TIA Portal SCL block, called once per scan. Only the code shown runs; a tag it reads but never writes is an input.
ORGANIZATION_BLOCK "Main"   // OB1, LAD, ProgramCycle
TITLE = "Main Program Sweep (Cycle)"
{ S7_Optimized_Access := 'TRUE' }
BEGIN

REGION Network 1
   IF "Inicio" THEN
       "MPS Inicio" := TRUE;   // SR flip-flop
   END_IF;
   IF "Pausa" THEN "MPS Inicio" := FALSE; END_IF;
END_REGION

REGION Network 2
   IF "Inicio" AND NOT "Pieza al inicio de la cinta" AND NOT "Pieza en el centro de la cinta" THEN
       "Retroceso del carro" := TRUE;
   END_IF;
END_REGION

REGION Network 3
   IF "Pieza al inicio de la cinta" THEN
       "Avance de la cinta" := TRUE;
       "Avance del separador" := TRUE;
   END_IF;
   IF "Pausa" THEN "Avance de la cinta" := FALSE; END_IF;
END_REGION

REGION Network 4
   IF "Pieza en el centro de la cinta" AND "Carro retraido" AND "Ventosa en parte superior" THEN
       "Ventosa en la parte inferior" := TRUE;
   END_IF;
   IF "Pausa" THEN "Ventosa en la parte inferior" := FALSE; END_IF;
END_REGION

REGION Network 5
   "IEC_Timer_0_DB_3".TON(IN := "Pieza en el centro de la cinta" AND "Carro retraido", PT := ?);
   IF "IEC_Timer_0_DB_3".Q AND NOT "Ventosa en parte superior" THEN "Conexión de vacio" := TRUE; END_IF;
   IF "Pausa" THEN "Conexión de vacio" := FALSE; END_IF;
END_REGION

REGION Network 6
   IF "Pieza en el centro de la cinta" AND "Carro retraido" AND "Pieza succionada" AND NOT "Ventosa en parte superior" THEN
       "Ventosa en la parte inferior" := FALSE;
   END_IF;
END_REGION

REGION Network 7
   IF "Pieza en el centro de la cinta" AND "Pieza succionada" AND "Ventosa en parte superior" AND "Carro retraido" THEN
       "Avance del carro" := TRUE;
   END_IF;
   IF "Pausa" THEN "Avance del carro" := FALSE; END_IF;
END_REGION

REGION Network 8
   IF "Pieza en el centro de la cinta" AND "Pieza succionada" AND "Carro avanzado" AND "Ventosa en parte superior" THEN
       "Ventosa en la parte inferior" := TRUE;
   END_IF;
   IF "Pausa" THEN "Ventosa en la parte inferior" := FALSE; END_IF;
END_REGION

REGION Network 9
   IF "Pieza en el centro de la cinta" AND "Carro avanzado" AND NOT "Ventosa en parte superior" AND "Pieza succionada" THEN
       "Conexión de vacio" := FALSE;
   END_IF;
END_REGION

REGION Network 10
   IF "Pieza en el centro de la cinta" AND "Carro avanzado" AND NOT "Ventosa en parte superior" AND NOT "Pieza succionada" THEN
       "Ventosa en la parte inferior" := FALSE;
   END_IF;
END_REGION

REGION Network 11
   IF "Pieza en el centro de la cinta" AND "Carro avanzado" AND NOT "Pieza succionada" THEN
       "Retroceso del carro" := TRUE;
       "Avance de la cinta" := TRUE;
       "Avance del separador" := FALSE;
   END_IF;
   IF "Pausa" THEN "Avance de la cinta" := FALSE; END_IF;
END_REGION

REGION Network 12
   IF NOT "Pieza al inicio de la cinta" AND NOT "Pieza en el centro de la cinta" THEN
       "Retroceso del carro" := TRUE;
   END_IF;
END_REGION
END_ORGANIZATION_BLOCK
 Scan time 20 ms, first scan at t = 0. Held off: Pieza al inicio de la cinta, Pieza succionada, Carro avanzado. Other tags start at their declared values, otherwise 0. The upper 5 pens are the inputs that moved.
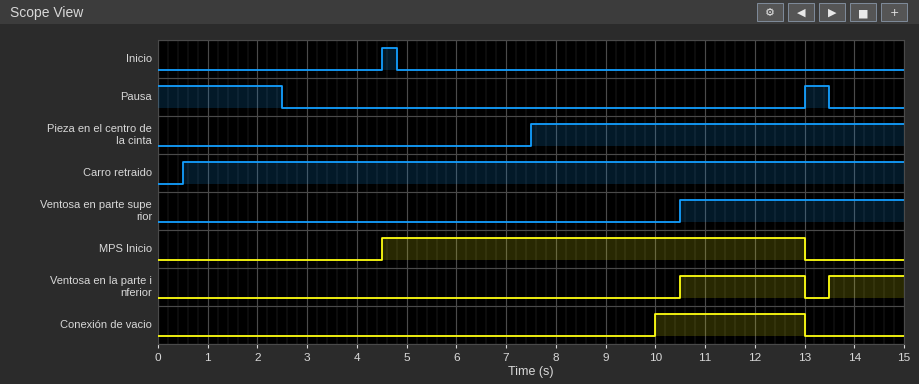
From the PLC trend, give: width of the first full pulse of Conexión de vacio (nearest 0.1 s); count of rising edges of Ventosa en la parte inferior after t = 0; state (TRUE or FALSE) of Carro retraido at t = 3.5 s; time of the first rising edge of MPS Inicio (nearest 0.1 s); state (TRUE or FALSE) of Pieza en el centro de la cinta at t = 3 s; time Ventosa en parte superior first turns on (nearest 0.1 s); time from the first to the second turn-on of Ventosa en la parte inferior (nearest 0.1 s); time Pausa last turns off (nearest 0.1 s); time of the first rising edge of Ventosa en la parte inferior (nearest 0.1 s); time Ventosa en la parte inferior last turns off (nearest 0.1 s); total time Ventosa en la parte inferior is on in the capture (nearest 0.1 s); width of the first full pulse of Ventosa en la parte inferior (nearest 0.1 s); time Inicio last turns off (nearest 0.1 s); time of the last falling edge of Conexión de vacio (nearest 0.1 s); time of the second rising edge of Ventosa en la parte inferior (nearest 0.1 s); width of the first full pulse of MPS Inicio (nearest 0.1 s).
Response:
3.0 s
2
TRUE
4.5 s
FALSE
10.5 s
3.0 s
13.5 s
10.5 s
13.0 s
4.0 s
2.5 s
4.8 s
13.0 s
13.5 s
8.5 s
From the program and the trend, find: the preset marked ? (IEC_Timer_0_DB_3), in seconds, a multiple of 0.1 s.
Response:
2.5 s
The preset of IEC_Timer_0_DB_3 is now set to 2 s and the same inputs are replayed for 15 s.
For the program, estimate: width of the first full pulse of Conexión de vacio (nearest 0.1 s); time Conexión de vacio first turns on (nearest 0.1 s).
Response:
3.5 s
9.5 s
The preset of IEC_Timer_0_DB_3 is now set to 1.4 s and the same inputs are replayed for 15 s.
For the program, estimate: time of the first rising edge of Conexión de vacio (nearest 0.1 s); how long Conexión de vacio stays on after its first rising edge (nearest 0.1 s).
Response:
8.9 s
4.1 s
